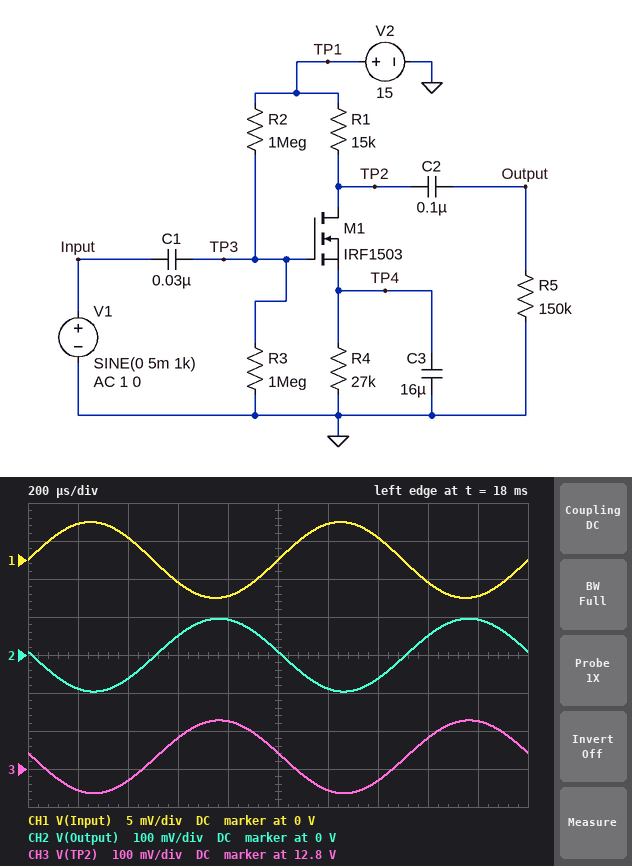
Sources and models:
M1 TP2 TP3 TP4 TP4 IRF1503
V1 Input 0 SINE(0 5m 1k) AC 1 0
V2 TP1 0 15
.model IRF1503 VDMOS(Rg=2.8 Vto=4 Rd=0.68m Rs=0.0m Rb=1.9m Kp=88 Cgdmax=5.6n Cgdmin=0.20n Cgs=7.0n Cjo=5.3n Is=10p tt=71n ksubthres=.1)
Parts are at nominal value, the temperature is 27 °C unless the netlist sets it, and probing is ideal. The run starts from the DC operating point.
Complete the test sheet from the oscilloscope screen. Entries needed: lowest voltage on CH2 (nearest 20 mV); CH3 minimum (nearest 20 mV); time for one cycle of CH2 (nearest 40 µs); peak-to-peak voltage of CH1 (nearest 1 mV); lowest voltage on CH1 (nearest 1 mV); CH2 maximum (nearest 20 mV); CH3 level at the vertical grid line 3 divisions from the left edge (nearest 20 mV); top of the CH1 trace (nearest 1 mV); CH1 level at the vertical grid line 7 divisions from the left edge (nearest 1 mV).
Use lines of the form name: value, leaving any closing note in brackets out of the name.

lowest voltage on CH2: -100 mV
CH3 minimum: 12.74 V
time for one cycle of CH2: 1.00 ms
peak-to-peak voltage of CH1: 10 mV
lowest voltage on CH1: -5 mV
CH2 maximum: 100 mV
CH3 level at the vertical grid line 3 divisions from the left edge: 12.88 V
top of the CH1 trace: 5 mV
CH1 level at the vertical grid line 7 divisions from the left edge: 3 mV
